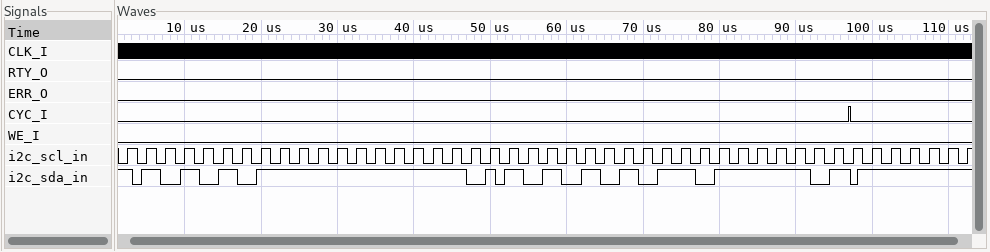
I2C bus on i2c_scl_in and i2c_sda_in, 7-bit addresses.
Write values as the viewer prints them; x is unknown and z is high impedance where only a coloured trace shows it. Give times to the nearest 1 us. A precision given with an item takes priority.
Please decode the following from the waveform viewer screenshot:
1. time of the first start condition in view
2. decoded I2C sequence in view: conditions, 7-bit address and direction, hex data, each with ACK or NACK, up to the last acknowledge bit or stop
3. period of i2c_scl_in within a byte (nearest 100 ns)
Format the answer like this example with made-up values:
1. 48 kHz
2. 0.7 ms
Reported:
1. 3 us
2. start, address 55 read NACK, FF ACK, repeated start, address 55 write NACK, BE NACK, stop
3. 2500 ns
